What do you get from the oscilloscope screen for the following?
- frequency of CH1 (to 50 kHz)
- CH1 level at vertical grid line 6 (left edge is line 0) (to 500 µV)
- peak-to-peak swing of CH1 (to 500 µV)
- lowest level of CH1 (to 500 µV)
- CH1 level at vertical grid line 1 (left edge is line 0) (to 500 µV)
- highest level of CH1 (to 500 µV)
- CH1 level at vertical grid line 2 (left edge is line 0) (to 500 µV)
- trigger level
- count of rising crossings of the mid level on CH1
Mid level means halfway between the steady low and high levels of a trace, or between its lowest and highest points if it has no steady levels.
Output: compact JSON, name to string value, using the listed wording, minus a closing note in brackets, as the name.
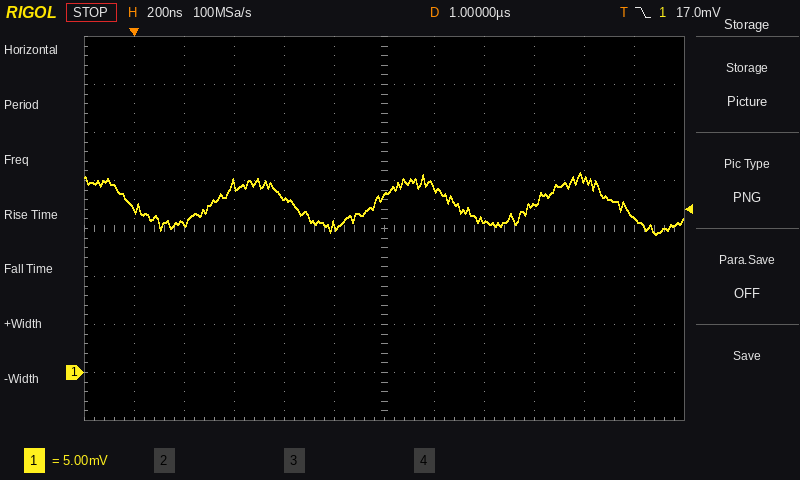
{"frequency of CH1": "1.55 MHz", "CH1 level at vertical grid line 6 (left edge is line 0)": "18.5 mV", "peak-to-peak swing of CH1": "6.5 mV", "lowest level of CH1": "14.5 mV", "CH1 level at vertical grid line 1 (left edge is line 0)": "17.0 mV", "highest level of CH1": "21.0 mV", "CH1 level at vertical grid line 2 (left edge is line 0)": "15.5 mV", "trigger level": "17.0 mV", "count of rising crossings of the mid level on CH1": "3"}
